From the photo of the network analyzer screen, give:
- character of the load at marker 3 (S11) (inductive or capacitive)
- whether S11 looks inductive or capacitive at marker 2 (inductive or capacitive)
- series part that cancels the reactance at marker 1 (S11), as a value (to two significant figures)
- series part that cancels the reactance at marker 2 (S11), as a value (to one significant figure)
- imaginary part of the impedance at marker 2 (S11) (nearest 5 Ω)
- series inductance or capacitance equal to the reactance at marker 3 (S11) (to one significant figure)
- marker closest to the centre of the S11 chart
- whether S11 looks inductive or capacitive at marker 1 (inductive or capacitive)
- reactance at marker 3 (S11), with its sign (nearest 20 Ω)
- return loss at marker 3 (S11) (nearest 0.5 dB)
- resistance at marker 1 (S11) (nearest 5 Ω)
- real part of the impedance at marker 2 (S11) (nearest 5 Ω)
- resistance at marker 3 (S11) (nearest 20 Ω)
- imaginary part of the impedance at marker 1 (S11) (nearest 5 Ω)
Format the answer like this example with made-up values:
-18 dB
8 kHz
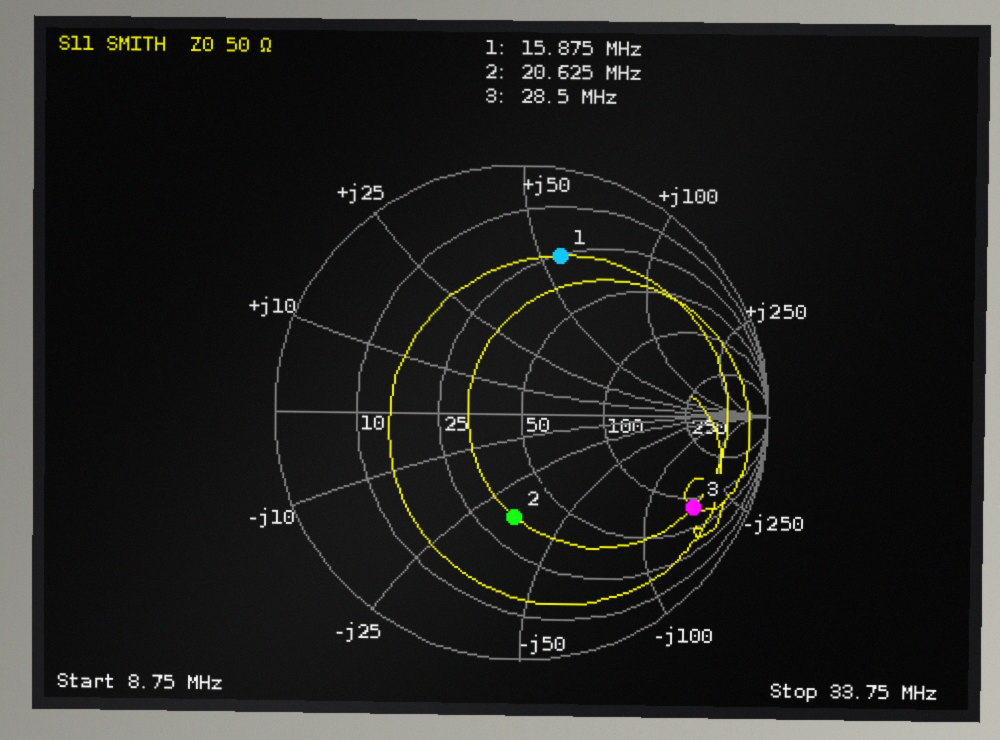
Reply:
capacitive
capacitive
180 pF
300 nH
-35 Ω
30 pF
marker 2
inductive
-160 Ω
2.0 dB
25 Ω
35 Ω
80 Ω
+55 Ω
